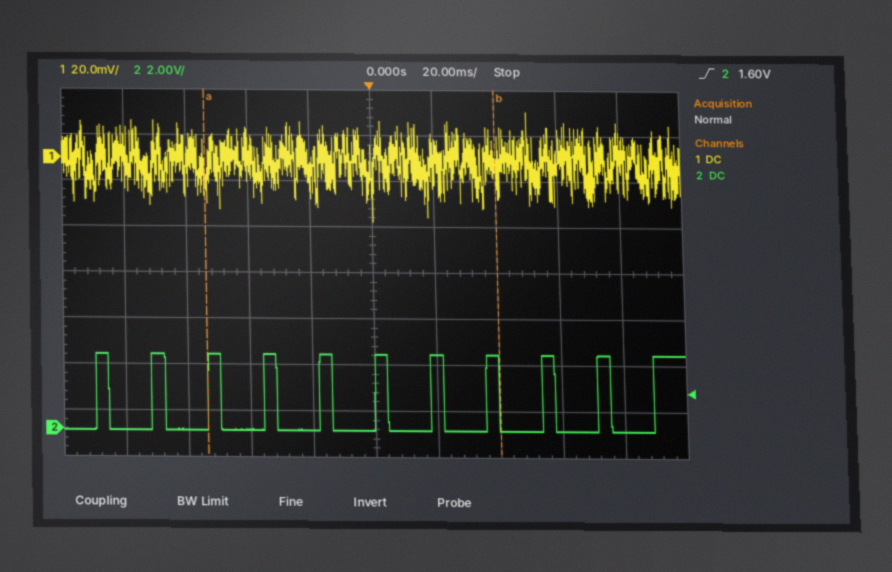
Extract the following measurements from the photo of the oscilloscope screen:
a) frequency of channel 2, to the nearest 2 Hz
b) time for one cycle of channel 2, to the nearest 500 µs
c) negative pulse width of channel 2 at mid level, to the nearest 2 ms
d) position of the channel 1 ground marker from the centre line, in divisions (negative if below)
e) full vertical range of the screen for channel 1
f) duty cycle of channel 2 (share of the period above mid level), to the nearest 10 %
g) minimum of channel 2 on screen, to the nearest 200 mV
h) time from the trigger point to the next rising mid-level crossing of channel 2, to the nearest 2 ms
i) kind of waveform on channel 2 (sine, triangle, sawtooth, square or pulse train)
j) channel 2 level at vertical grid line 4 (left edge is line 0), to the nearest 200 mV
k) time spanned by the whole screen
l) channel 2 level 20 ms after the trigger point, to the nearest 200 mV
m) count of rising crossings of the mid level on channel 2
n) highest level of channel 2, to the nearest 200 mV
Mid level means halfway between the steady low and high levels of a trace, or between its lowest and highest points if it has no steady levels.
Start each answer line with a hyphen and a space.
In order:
- 56 Hz
- 18.0 ms
- 14 ms
- +2.5 div
- 160 mV
- 20 %
- 0.0 V
- 18 ms
- pulse train
- 0.0 V
- 200 ms
- 3.2 V
- 11
- 3.2 V
